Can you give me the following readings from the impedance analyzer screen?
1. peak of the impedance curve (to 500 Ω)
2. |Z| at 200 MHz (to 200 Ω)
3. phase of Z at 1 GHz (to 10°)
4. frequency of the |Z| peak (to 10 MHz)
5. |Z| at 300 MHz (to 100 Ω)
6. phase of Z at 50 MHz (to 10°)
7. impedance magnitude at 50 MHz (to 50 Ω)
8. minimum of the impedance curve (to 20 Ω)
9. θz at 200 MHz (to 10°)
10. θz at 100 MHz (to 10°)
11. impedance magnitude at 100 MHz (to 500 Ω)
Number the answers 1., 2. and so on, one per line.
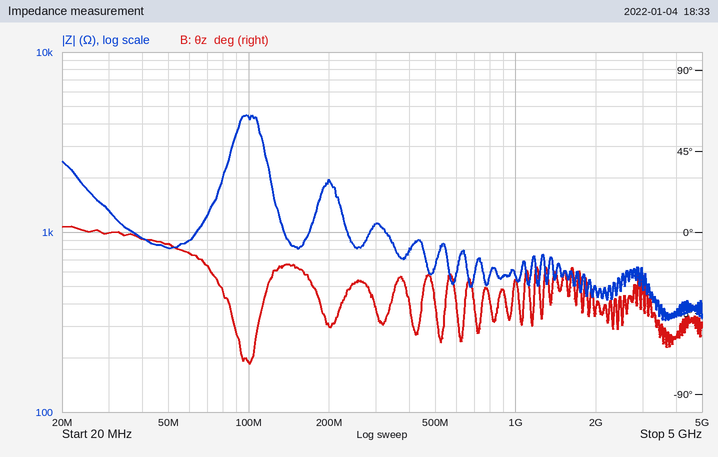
1. 4.5 kΩ
2. 2.0 kΩ
3. -30°
4. 100 MHz
5. 1.1 kΩ
6. -10°
7. 800 Ω
8. 320 Ω
9. -50°
10. -70°
11. 4.5 kΩ
